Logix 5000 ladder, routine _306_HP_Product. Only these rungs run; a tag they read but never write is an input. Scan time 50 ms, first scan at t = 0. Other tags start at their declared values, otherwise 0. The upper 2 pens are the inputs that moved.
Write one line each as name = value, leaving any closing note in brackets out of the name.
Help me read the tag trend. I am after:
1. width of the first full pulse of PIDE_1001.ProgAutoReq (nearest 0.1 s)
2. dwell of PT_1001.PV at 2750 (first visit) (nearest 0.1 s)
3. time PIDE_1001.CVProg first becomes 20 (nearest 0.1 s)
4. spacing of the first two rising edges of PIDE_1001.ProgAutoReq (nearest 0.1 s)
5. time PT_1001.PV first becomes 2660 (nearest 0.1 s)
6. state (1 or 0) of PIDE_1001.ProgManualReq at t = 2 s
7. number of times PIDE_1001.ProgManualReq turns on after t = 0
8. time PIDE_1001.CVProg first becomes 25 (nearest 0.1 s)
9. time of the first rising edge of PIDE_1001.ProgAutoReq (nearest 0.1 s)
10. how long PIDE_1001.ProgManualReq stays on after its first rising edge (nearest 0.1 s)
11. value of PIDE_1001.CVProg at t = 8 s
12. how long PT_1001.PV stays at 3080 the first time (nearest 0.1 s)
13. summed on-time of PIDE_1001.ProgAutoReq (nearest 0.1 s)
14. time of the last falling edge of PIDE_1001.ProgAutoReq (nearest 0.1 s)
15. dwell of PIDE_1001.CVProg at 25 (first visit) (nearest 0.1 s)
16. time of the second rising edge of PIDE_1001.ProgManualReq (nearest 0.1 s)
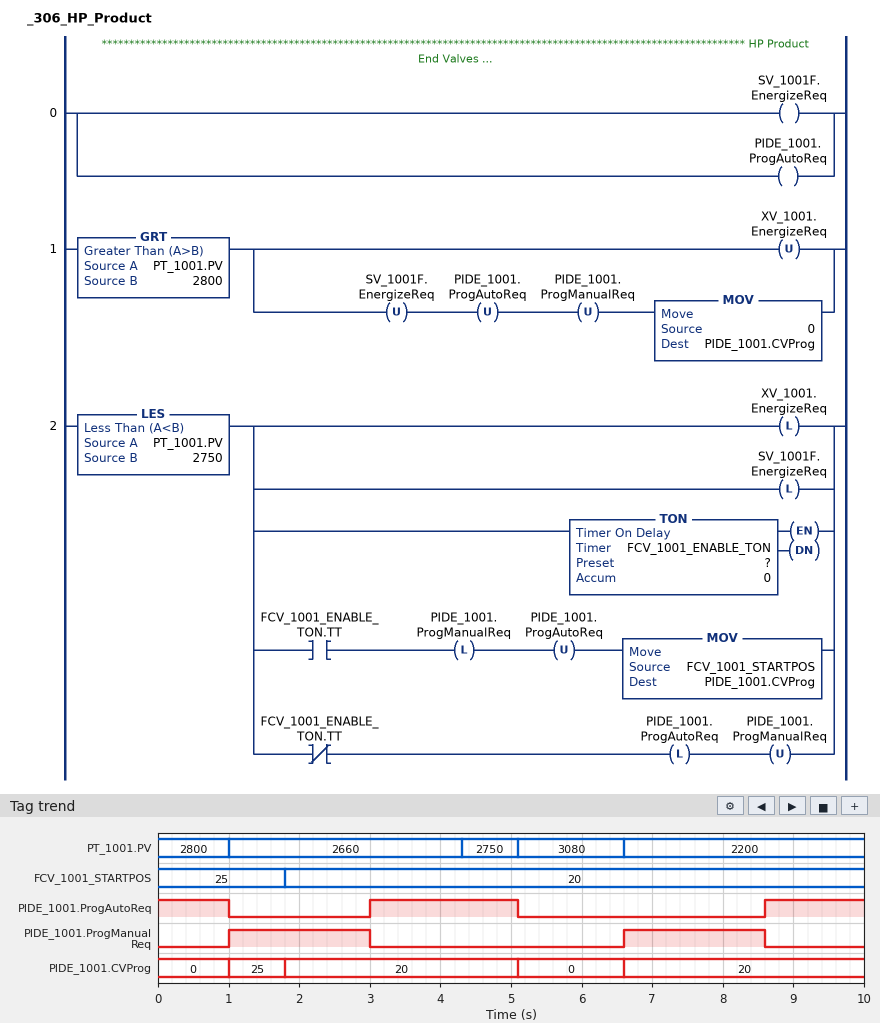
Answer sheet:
width of the first full pulse of PIDE_1001.ProgAutoReq = 2.1 s
dwell of PT_1001.PV at 2750 (first visit) = 0.8 s
time PIDE_1001.CVProg first becomes 20 = 1.8 s
spacing of the first two rising edges of PIDE_1001.ProgAutoReq = 5.6 s
time PT_1001.PV first becomes 2660 = 1.0 s
state (1 or 0) of PIDE_1001.ProgManualReq at t = 2 s = 1
number of times PIDE_1001.ProgManualReq turns on after t = 0 = 2
time PIDE_1001.CVProg first becomes 25 = 1.0 s
time of the first rising edge of PIDE_1001.ProgAutoReq = 3.0 s
how long PIDE_1001.ProgManualReq stays on after its first rising edge = 2.0 s
value of PIDE_1001.CVProg at t = 8 s = 20
how long PT_1001.PV stays at 3080 the first time = 1.5 s
summed on-time of PIDE_1001.ProgAutoReq = 4.5 s
time of the last falling edge of PIDE_1001.ProgAutoReq = 5.1 s
dwell of PIDE_1001.CVProg at 25 (first visit) = 0.8 s
time of the second rising edge of PIDE_1001.ProgManualReq = 6.6 s
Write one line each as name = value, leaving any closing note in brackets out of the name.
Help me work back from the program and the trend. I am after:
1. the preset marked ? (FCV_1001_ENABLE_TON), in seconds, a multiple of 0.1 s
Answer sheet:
the preset marked ? (FCV_1001_ENABLE_TON), in seconds, a multiple of 0.1 s = 2.0 s
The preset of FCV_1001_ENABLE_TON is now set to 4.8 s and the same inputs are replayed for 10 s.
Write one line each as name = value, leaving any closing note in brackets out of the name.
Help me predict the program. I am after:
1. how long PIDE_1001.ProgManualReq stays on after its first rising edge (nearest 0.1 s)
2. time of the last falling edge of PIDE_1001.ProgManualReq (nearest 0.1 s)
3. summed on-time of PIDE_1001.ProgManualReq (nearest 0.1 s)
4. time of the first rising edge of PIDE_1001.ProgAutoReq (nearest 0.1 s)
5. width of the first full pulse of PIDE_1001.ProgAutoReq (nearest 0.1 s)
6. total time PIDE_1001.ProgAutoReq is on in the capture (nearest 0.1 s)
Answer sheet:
how long PIDE_1001.ProgManualReq stays on after its first rising edge = 4.1 s
time of the last falling edge of PIDE_1001.ProgManualReq = 5.1 s
summed on-time of PIDE_1001.ProgManualReq = 7.5 s
time of the first rising edge of PIDE_1001.ProgAutoReq = 4.3 s
width of the first full pulse of PIDE_1001.ProgAutoReq = 0.8 s
total time PIDE_1001.ProgAutoReq is on in the capture = 1.8 s
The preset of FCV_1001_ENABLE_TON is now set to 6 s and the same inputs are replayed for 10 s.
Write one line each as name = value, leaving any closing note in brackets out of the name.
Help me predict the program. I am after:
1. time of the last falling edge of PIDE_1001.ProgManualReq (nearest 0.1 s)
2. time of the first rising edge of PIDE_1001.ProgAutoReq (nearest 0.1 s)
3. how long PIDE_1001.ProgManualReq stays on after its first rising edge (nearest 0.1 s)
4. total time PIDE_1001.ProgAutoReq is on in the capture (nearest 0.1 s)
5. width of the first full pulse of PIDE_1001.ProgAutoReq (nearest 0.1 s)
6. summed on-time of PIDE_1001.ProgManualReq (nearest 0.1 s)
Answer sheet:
time of the last falling edge of PIDE_1001.ProgManualReq = 5.1 s
time of the first rising edge of PIDE_1001.ProgAutoReq = 4.3 s
how long PIDE_1001.ProgManualReq stays on after its first rising edge = 4.1 s
total time PIDE_1001.ProgAutoReq is on in the capture = 1.8 s
width of the first full pulse of PIDE_1001.ProgAutoReq = 0.8 s
summed on-time of PIDE_1001.ProgManualReq = 7.5 s
